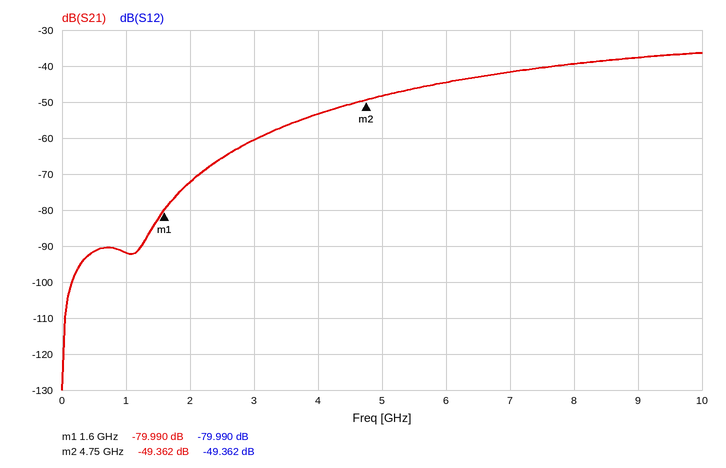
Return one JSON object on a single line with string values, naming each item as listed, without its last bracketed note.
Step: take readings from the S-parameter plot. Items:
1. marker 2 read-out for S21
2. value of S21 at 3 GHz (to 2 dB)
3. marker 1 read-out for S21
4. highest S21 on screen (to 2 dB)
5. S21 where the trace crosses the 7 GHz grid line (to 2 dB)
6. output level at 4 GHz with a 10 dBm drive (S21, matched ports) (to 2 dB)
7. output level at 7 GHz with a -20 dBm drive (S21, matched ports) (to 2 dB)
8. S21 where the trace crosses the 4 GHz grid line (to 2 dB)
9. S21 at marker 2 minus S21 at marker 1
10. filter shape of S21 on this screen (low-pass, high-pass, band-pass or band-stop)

{"marker 2 read-out for S21": "-49.362 dB", "value of S21 at 3 GHz": "-60 dB", "marker 1 read-out for S21": "-79.990 dB", "highest S21 on screen": "-36 dB", "S21 where the trace crosses the 7 GHz grid line": "-42 dB", "output level at 4 GHz with a 10 dBm drive (S21, matched ports)": "-44 dBm", "output level at 7 GHz with a -20 dBm drive (S21, matched ports)": "-62 dBm", "S21 where the trace crosses the 4 GHz grid line": "-54 dB", "S21 at marker 2 minus S21 at marker 1": "30.628 dB", "filter shape of S21 on this screen": "high-pass"}
